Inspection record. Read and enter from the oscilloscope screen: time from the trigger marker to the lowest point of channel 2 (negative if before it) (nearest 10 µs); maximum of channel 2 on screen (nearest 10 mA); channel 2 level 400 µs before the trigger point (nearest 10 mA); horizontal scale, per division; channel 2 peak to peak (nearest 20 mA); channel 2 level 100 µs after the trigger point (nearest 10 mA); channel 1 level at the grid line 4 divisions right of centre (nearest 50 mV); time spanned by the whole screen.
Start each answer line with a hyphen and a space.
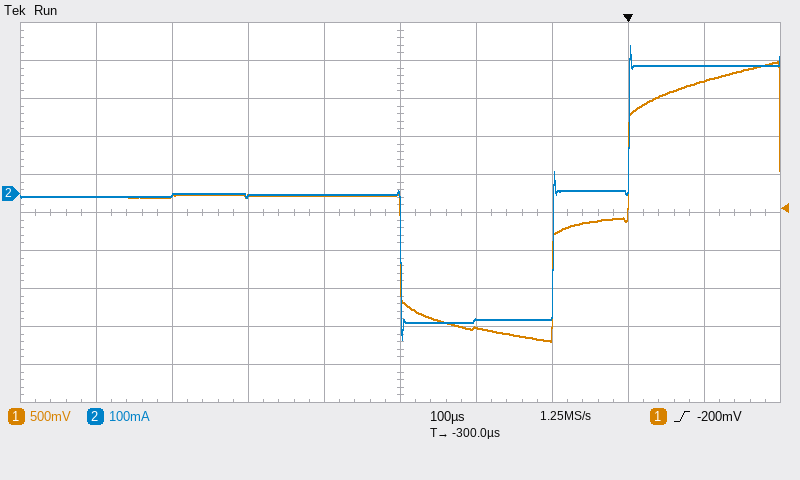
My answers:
- -300 µs
- 390 mA
- 0 mA
- 100 µs
- 780 mA
- 340 mA
- 1.50 V
- 1 ms
